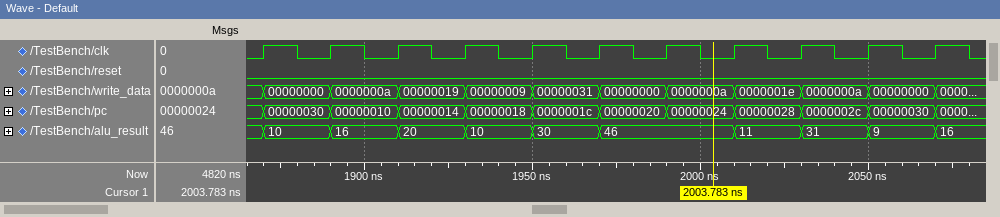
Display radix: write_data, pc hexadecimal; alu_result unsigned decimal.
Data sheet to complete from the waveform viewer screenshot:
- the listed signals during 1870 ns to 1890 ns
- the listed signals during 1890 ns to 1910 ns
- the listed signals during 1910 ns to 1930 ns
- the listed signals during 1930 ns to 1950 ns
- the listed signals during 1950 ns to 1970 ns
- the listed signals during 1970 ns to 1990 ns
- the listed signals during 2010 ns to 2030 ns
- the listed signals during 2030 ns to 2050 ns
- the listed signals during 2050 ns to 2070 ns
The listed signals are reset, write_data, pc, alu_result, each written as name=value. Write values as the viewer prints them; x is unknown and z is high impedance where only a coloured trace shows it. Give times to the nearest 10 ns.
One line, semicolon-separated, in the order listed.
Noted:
reset=0, write_data=00000000, pc=00000030, alu_result=10; reset=0, write_data=0000000a, pc=00000010, alu_result=16; reset=0, write_data=00000019, pc=00000014, alu_result=20; reset=0, write_data=00000009, pc=00000018, alu_result=10; reset=0, write_data=00000031, pc=0000001c, alu_result=30; reset=0, write_data=00000000, pc=00000020, alu_result=46; reset=0, write_data=0000001e, pc=00000028, alu_result=11; reset=0, write_data=0000000a, pc=0000002c, alu_result=31; reset=0, write_data=00000000, pc=00000030, alu_result=9
